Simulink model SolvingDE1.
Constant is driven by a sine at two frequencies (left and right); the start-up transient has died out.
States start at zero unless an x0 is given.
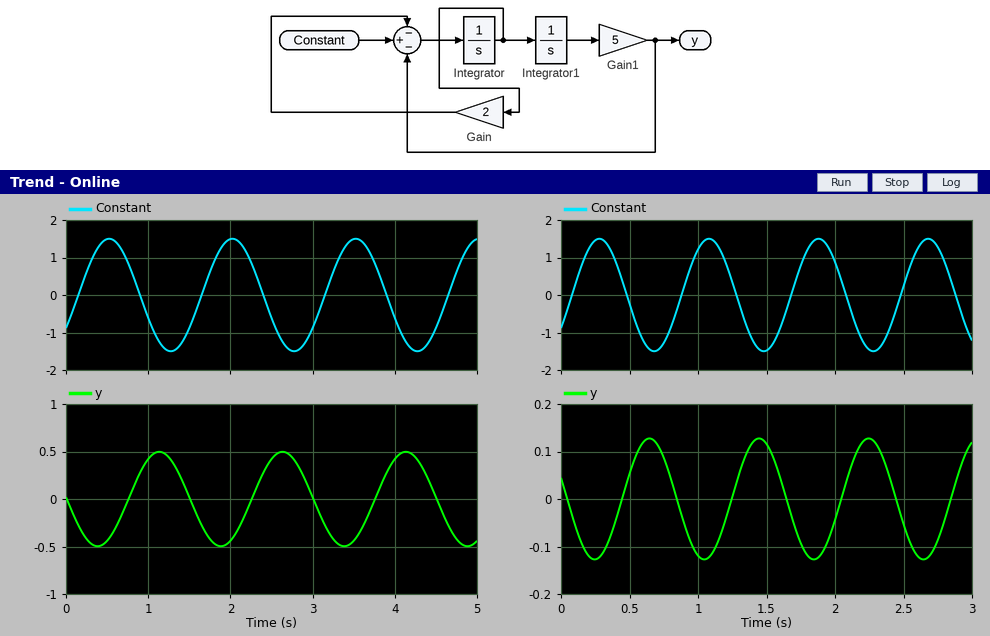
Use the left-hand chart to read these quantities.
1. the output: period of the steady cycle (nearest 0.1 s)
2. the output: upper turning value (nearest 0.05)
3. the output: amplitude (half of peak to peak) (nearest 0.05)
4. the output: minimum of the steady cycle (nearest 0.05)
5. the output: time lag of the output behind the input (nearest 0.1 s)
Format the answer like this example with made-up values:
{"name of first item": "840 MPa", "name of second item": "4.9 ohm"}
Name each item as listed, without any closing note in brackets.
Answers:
{"the output: period of the steady cycle": "1.5 s", "the output: upper turning value": "0.50", "the output: amplitude (half of peak to peak)": "0.50", "the output: minimum of the steady cycle": "-0.50", "the output: time lag of the output behind the input": "0.6 s"}
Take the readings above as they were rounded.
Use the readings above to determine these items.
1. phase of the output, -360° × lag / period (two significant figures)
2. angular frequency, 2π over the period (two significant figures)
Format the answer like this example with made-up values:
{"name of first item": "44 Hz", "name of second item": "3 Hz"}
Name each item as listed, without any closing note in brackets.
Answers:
{"phase of the output, -360° × lag / period": "-140°", "angular frequency, 2π over the period": "4.2 rad/s"}
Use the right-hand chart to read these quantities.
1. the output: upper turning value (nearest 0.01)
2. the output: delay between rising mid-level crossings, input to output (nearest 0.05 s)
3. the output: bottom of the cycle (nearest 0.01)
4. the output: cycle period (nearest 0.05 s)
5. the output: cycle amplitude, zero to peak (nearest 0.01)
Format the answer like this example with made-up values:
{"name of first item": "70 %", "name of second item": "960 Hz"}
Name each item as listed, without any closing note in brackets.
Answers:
{"the output: upper turning value": "0.13", "the output: delay between rising mid-level crossings, input to output": "0.35 s", "the output: bottom of the cycle": "-0.13", "the output: cycle period": "0.80 s", "the output: cycle amplitude, zero to peak": "0.13"}
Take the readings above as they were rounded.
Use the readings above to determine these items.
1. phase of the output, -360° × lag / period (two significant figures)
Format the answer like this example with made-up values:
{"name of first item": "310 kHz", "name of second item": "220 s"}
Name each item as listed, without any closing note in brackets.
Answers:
{"phase of the output, -360° × lag / period": "-160°"}
